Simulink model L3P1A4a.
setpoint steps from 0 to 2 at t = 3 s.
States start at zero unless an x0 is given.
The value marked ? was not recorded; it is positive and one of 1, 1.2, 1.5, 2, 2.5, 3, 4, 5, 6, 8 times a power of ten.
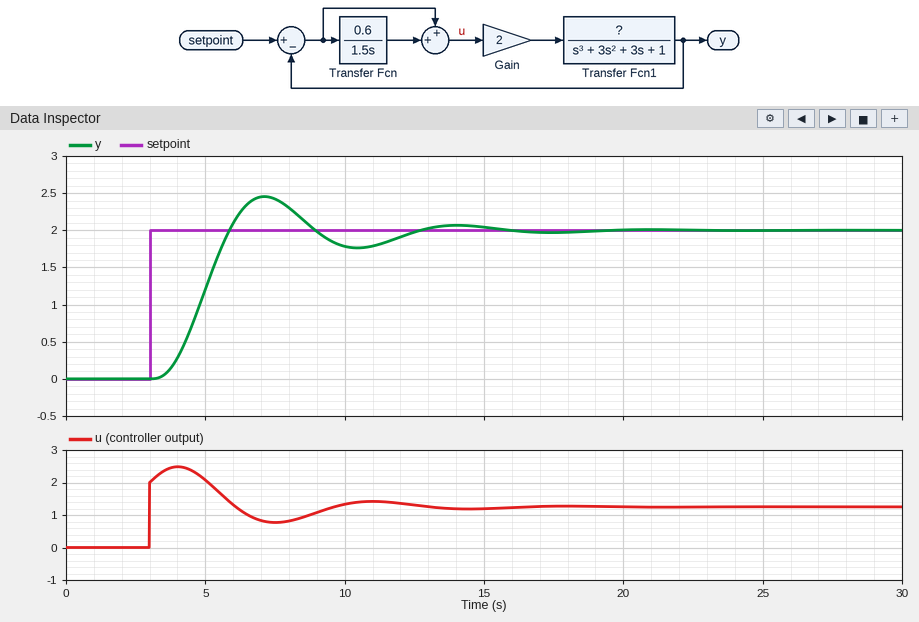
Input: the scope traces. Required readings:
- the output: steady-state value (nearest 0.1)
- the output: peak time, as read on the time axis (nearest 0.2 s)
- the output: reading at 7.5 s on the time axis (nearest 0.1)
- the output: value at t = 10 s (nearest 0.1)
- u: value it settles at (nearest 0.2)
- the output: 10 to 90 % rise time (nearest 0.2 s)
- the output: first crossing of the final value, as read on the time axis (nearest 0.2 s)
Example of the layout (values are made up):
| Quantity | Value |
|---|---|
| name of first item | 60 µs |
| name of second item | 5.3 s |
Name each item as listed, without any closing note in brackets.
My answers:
| Quantity | Value |
|---|---|
| the output: steady-state value | 2.0 |
| the output: peak time, as read on the time axis | 7.2 s |
| the output: reading at 7.5 s on the time axis | 2.4 |
| the output: value at t = 10 s | 1.8 |
| u: value it settles at | 1.2 |
| the output: 10 to 90 % rise time | 1.8 s |
| the output: first crossing of the final value, as read on the time axis | 5.8 s |
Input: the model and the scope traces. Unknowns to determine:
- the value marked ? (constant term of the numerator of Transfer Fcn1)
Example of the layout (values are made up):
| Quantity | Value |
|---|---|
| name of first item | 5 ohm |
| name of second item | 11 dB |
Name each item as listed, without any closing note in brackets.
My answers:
| Quantity | Value |
|---|---|
| the value marked ? | 0.8 |
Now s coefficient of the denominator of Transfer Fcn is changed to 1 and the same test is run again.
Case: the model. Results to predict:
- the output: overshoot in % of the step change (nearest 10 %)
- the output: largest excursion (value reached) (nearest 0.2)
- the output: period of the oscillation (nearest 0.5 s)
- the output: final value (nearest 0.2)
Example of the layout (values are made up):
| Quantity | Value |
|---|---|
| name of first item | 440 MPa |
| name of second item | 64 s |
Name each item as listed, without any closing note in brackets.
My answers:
| Quantity | Value |
|---|---|
| the output: overshoot in % of the step change | 40 % |
| the output: largest excursion (value reached) | 2.8 |
| the output: period of the oscillation | 7.0 s |
| the output: final value | 2.0 |
